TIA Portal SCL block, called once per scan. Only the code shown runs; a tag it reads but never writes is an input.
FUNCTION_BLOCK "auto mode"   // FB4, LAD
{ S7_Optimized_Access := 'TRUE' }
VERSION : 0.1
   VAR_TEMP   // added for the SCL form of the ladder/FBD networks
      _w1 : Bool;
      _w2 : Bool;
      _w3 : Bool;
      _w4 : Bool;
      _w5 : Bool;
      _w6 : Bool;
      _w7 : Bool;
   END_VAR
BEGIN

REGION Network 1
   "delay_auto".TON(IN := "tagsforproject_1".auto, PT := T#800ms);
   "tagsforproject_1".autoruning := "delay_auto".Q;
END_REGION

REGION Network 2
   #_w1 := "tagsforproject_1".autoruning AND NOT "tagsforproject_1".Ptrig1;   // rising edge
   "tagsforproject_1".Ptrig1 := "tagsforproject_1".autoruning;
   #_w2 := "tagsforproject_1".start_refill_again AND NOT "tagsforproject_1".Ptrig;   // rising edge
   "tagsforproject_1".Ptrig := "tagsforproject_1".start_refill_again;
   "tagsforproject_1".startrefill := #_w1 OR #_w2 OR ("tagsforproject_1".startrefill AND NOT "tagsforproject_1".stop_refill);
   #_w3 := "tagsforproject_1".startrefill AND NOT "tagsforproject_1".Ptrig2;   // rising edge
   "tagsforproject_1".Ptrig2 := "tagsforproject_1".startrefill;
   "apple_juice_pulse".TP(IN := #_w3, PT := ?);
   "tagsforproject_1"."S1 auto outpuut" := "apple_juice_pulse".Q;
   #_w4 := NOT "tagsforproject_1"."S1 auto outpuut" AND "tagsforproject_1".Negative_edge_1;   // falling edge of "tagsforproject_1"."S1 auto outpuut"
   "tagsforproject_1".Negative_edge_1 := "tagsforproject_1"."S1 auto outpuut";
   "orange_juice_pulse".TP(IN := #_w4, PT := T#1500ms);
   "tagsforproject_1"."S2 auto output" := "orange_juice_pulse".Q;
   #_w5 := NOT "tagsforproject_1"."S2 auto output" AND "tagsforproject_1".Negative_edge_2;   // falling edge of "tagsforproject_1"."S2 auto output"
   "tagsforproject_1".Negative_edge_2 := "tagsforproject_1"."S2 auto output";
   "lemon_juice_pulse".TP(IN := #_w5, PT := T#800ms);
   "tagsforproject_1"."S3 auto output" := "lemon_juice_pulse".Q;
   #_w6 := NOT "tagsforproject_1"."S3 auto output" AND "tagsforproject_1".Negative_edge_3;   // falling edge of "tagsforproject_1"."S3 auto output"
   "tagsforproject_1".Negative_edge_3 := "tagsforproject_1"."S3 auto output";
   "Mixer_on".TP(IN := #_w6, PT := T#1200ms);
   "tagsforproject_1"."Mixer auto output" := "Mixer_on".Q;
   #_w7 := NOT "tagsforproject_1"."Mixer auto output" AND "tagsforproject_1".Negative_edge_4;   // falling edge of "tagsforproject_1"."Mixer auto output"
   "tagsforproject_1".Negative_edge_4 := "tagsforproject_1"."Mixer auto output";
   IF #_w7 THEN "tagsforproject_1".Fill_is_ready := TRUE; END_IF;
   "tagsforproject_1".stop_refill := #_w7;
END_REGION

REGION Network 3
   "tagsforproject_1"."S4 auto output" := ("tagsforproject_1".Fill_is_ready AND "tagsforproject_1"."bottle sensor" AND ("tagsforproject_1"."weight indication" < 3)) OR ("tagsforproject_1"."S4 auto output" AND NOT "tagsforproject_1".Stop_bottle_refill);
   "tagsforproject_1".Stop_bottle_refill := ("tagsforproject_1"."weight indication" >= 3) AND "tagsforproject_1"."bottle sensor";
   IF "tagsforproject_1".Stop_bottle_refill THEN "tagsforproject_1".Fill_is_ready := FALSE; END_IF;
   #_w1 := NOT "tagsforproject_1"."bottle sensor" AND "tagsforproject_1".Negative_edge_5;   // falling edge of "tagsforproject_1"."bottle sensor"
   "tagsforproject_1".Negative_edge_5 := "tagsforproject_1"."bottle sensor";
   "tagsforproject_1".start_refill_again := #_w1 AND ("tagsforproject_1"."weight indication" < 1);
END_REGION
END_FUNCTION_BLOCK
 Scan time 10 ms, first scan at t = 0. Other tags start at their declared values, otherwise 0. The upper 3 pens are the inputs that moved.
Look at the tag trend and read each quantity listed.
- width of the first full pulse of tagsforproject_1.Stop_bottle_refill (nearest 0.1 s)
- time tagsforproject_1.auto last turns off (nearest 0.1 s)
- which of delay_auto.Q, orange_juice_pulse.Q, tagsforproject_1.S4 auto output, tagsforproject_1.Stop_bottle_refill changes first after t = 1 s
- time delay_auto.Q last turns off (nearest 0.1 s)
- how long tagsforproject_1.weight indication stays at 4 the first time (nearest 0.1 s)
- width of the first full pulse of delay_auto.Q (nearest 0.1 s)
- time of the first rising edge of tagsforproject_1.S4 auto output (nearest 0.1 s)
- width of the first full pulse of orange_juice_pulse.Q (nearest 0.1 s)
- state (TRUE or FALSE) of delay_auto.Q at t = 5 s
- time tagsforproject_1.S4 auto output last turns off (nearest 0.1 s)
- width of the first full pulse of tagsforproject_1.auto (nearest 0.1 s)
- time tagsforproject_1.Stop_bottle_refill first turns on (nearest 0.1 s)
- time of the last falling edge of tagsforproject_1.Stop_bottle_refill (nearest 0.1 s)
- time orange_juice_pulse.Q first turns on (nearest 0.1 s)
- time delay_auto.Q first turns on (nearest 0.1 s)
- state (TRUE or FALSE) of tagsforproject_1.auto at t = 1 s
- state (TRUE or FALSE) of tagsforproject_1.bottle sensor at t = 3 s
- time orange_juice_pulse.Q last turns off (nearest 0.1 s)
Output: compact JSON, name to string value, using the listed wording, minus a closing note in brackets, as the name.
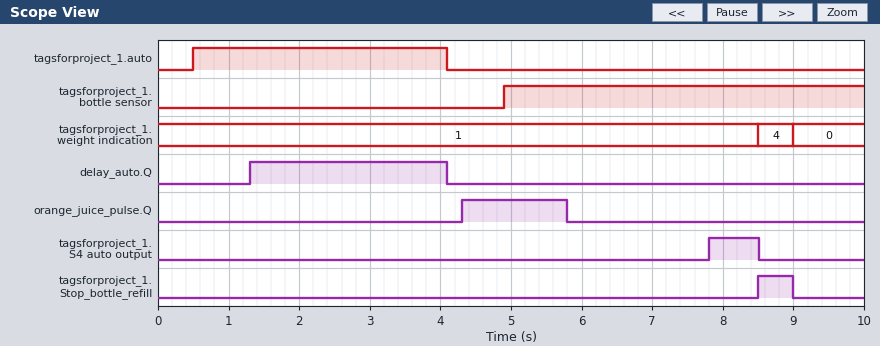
{"width of the first full pulse of tagsforproject_1.Stop_bottle_refill": "0.5 s", "time tagsforproject_1.auto last turns off": "4.1 s", "which of delay_auto.Q, orange_juice_pulse.Q, tagsforproject_1.S4 auto output, tagsforproject_1.Stop_bottle_refill changes first after t = 1 s": "delay_auto.Q", "time delay_auto.Q last turns off": "4.1 s", "how long tagsforproject_1.weight indication stays at 4 the first time": "0.5 s", "width of the first full pulse of delay_auto.Q": "2.8 s", "time of the first rising edge of tagsforproject_1.S4 auto output": "7.8 s", "width of the first full pulse of orange_juice_pulse.Q": "1.5 s", "state (TRUE or FALSE) of delay_auto.Q at t = 5 s": "FALSE", "time tagsforproject_1.S4 auto output last turns off": "8.5 s", "width of the first full pulse of tagsforproject_1.auto": "3.6 s", "time tagsforproject_1.Stop_bottle_refill first turns on": "8.5 s", "time of the last falling edge of tagsforproject_1.Stop_bottle_refill": "9.0 s", "time orange_juice_pulse.Q first turns on": "4.3 s", "time delay_auto.Q first turns on": "1.3 s", "state (TRUE or FALSE) of tagsforproject_1.auto at t = 1 s": "TRUE", "state (TRUE or FALSE) of tagsforproject_1.bottle sensor at t = 3 s": "FALSE", "time orange_juice_pulse.Q last turns off": "5.8 s"}
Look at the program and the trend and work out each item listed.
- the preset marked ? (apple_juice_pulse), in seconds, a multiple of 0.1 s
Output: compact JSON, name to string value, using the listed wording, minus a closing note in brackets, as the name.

{"the preset marked ? (apple_juice_pulse), in seconds, a multiple of 0.1 s": "3.0 s"}
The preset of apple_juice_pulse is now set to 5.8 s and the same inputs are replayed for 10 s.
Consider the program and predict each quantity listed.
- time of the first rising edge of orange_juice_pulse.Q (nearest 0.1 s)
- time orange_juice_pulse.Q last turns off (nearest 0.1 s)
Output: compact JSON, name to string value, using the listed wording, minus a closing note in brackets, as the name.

{"time of the first rising edge of orange_juice_pulse.Q": "7.1 s", "time orange_juice_pulse.Q last turns off": "8.6 s"}
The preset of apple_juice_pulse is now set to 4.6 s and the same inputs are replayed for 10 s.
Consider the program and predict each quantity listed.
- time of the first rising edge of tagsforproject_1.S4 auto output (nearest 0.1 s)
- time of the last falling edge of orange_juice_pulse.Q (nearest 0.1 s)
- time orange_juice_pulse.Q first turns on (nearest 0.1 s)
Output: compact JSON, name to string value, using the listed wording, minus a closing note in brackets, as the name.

{"time of the first rising edge of tagsforproject_1.S4 auto output": "9.4 s", "time of the last falling edge of orange_juice_pulse.Q": "7.4 s", "time orange_juice_pulse.Q first turns on": "5.9 s"}
